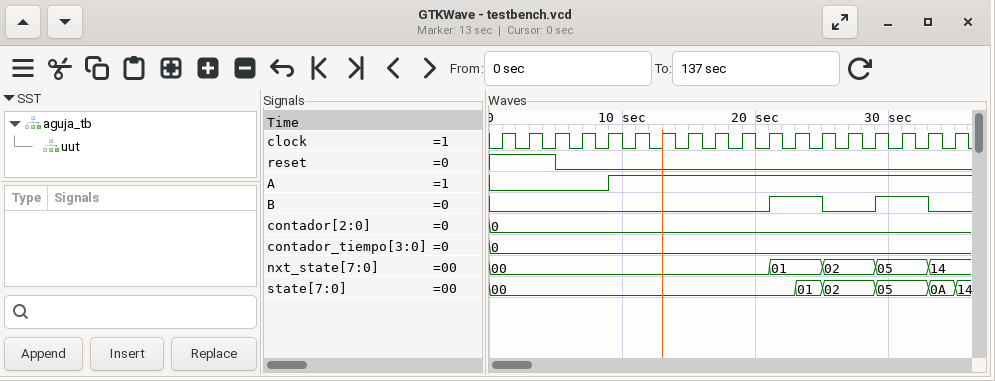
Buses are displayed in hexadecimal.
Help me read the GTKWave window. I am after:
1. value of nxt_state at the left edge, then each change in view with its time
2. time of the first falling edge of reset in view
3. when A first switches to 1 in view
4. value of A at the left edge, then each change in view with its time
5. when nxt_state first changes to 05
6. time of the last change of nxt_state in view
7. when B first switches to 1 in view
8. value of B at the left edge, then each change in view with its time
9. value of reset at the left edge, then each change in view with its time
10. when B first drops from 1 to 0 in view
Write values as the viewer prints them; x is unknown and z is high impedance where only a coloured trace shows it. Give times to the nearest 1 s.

00, 01 at 21 s, 02 at 25 s, 05 at 29 s, 14 at 33 s
5 s
9 s
0, 1 at 9 s
29 s
33 s
21 s
0, 1 at 21 s, 0 at 25 s, 1 at 29 s, 0 at 33 s
1, 0 at 5 s
25 s
